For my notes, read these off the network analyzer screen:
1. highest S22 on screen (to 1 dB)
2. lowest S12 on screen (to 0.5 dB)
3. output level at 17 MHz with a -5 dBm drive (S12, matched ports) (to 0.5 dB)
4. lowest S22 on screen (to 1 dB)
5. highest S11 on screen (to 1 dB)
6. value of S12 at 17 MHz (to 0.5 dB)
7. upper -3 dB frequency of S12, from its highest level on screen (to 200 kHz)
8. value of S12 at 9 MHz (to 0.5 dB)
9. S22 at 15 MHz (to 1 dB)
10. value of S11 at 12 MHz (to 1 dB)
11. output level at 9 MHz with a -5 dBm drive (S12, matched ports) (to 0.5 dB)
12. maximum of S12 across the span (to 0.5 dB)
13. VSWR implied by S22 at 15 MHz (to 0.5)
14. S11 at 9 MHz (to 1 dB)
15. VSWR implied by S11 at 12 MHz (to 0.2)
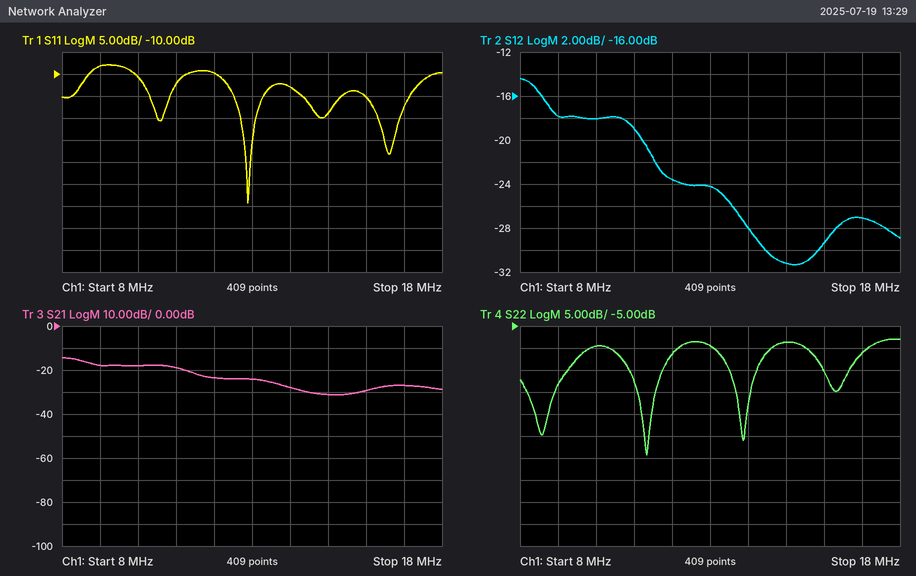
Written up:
-8 dB
-31.5 dB
-32.0 dBm
-34 dB
-8 dB
-27.0 dB
8.8 MHz
-18.0 dB
-9 dB
-10 dB
-23.0 dBm
-14.5 dB
2.0
-8 dB
2.0
